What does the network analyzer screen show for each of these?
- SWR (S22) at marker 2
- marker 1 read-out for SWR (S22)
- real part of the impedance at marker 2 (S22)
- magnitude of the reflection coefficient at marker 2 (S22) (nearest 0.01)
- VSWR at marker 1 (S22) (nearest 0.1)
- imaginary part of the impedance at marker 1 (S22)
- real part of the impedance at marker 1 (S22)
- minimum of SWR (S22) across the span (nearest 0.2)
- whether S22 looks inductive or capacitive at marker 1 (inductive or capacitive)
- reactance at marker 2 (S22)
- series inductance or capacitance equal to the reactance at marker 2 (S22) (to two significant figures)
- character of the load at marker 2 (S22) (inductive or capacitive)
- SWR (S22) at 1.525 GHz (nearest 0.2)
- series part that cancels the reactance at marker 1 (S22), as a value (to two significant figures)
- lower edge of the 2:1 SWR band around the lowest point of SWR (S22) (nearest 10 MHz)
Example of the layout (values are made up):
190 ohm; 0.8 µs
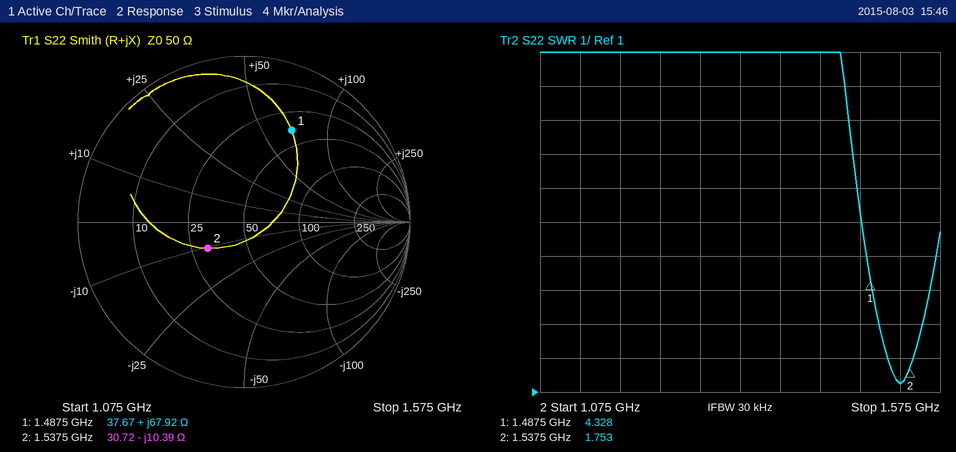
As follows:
1.753; 4.328; 30.72 Ω; 0.27; 4.3; +67.92 Ω; 37.67 Ω; 1.2; inductive; -10.39 Ω; 10.0 pF; capacitive; 1.2; 1.6 pF; 1.51 GHz
